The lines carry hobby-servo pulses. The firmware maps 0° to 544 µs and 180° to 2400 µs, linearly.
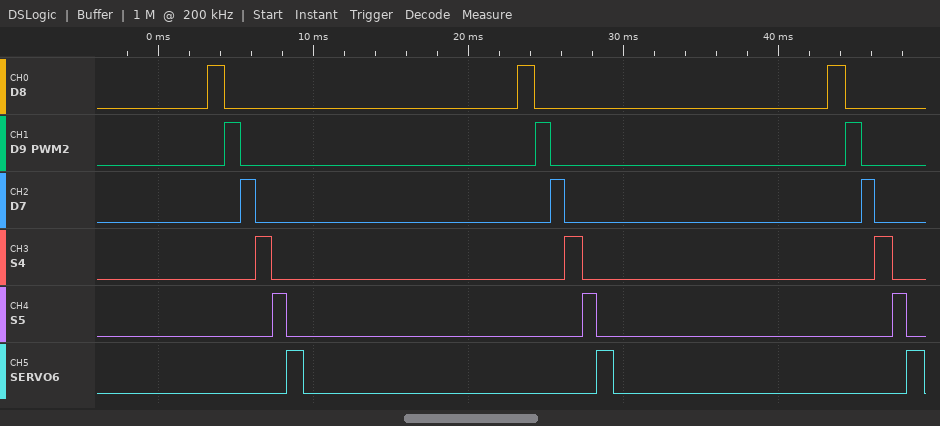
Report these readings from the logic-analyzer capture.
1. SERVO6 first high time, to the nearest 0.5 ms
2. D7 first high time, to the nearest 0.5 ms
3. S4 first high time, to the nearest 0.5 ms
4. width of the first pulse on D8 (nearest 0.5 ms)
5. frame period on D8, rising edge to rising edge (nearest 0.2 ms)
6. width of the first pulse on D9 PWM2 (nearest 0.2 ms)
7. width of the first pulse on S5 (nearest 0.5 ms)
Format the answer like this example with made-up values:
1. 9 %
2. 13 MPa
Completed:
1. 1.0 ms
2. 1.0 ms
3. 1.0 ms
4. 1.0 ms
5. 20.0 ms
6. 1.0 ms
7. 1.0 ms
